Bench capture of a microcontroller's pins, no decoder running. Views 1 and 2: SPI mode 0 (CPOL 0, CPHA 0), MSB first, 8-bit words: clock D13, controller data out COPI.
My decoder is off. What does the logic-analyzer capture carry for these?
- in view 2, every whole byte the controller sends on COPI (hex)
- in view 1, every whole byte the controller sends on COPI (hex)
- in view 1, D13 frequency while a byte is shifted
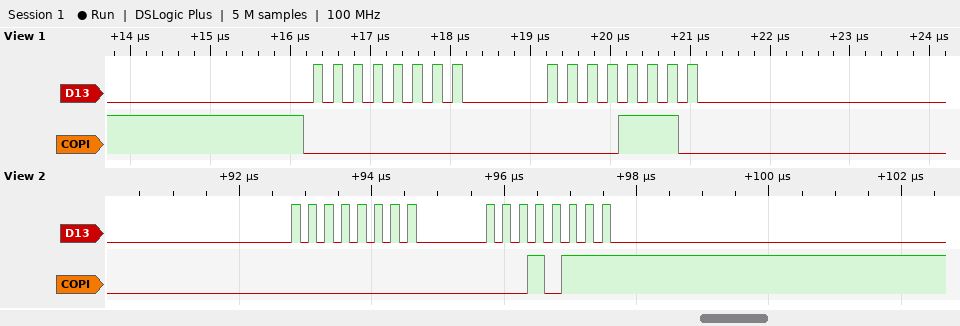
00 17
00 0E
4 MHz
